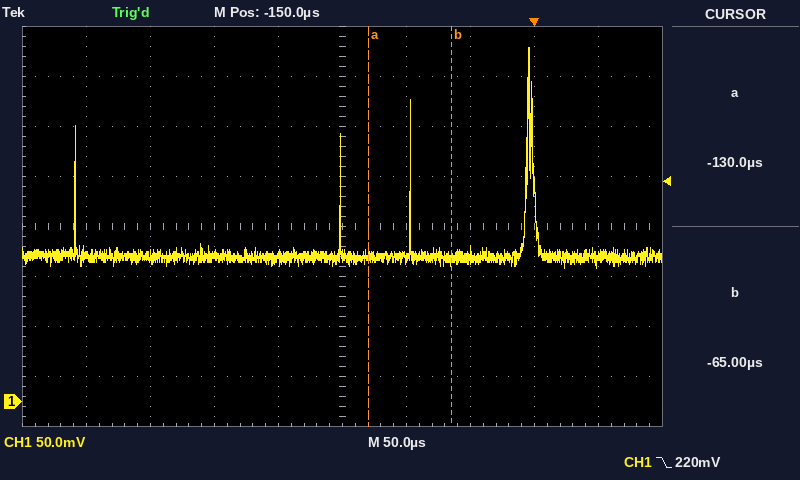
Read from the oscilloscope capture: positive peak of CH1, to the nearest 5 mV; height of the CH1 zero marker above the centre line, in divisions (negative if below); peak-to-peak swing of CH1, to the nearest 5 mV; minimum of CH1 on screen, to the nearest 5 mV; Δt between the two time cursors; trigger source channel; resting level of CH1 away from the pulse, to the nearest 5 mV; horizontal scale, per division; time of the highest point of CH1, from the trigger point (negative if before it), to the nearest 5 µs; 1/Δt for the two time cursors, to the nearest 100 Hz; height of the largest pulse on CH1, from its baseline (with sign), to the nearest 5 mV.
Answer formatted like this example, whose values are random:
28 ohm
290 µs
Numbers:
355 mV
-3.5 div
220 mV
135 mV
65 µs
CH1
145 mV
50 µs
-5 µs
15.4 kHz
+210 mV
